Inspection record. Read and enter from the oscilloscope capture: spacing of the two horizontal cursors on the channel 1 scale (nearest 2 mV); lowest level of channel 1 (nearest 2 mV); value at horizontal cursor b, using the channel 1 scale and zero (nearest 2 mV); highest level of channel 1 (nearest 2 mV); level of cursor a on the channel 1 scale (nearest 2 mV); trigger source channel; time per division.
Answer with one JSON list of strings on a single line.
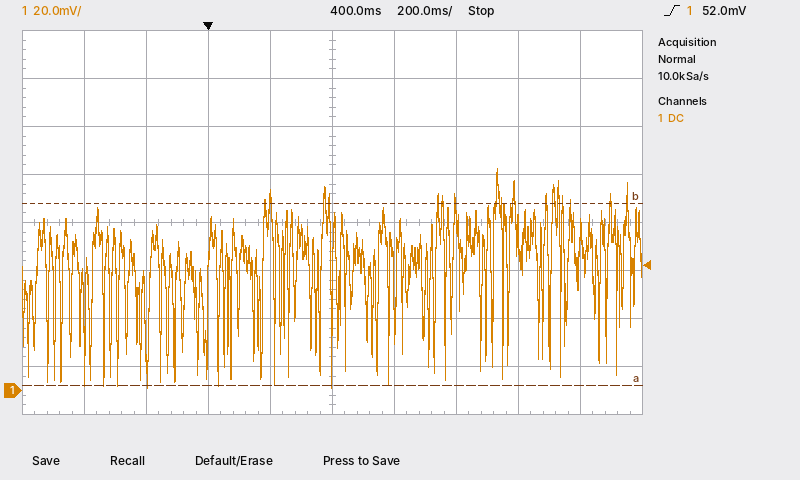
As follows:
["76 mV", "2 mV", "78 mV", "92 mV", "2 mV", "channel 1", "200 ms"]
